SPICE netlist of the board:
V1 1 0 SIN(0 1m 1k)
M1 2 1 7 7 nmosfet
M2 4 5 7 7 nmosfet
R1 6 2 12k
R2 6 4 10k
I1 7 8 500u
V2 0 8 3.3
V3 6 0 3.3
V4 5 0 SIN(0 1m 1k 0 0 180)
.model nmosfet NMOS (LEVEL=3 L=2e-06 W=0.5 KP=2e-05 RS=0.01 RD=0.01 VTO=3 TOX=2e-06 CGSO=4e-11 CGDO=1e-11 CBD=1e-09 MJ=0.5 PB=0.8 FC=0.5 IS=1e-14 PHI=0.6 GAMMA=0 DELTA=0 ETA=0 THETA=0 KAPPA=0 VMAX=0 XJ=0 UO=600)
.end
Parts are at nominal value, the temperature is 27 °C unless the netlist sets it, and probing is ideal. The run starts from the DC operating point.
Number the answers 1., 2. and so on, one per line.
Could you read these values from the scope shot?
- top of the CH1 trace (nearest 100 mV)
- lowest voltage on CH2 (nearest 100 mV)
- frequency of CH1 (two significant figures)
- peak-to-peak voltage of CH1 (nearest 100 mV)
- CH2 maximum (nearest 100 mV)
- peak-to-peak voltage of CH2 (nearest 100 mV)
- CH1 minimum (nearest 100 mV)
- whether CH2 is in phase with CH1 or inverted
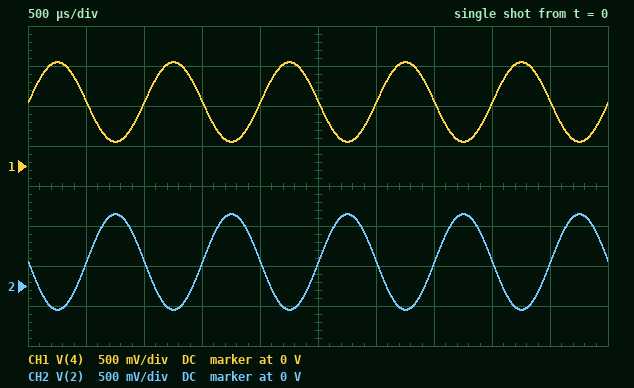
1. 1.3 V
2. -300 mV
3. 1.0 kHz
4. 1.0 V
5. 900 mV
6. 1.2 V
7. 300 mV
8. inverted
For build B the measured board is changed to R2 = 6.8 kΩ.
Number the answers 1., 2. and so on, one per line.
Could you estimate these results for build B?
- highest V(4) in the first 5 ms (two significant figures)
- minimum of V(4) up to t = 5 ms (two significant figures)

1. 1.9 V
2. 1.3 V
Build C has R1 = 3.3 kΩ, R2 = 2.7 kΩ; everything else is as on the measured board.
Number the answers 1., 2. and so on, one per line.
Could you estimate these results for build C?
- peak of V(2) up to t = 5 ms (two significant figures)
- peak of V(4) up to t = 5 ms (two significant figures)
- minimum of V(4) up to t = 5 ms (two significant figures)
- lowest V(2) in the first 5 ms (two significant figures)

1. 2.6 V
2. 2.8 V
3. 2.5 V
4. 2.3 V
